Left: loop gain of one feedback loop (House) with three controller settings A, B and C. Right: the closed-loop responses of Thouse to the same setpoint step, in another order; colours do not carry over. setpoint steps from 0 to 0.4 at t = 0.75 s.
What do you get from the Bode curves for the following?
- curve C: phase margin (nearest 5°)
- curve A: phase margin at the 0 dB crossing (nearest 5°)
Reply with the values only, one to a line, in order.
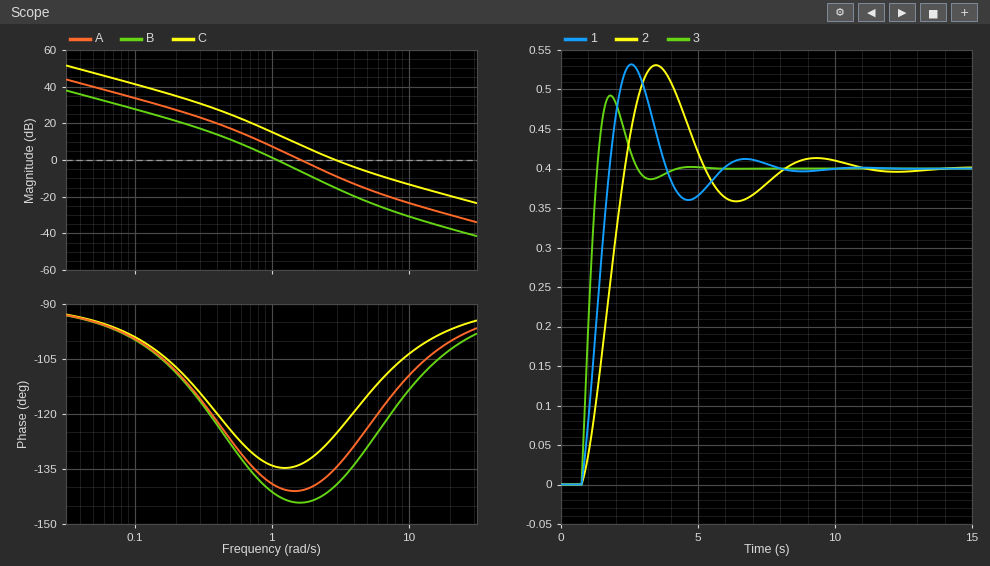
55°
40°
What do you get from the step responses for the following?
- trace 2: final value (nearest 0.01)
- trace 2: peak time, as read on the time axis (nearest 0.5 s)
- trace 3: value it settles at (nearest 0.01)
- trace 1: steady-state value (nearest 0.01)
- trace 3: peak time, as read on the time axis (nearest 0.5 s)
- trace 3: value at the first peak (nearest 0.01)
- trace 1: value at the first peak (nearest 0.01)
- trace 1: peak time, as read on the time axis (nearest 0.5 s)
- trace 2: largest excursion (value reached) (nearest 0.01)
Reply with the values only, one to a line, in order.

0.40
3.5 s
0.40
0.40
2.0 s
0.49
0.53
2.5 s
0.53
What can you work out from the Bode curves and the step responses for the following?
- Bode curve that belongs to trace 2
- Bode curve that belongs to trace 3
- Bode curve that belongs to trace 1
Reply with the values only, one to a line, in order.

B
C
A
